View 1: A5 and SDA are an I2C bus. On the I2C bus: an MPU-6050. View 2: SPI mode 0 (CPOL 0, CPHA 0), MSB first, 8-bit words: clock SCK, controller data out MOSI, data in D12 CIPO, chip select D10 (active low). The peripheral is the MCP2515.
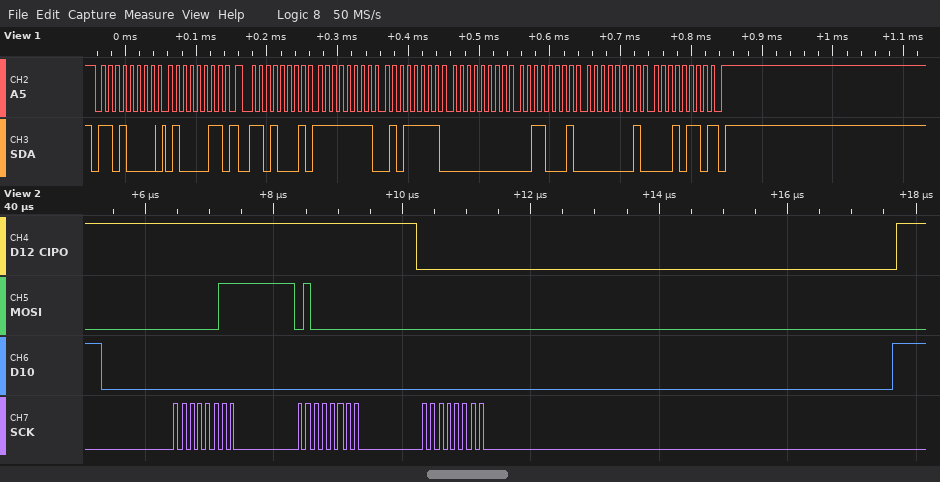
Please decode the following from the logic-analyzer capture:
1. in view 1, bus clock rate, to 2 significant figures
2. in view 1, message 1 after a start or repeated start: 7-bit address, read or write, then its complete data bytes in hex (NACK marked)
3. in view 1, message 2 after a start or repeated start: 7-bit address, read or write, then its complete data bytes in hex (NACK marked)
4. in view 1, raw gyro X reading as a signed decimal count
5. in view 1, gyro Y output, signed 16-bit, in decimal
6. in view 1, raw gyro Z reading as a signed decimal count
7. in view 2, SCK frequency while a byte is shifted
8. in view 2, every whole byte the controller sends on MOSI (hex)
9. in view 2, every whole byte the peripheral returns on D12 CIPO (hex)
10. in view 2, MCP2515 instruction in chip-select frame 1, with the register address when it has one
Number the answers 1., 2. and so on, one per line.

1. 100 kHz
2. 0x68 write: 43
3. 0x68 read: FF 5F 00 31 01 16 NACK
4. -161
5. 49
6. 278
7. 8 MHz
8. 03 40 00
9. FF FF 00
10. READ 0x40
